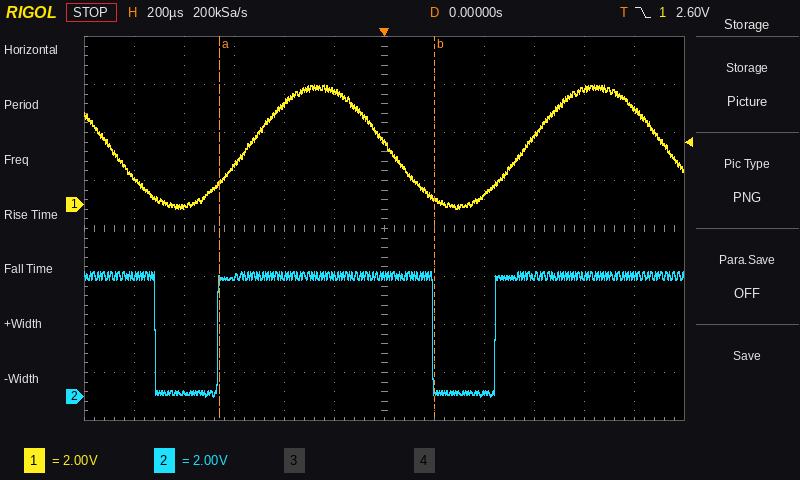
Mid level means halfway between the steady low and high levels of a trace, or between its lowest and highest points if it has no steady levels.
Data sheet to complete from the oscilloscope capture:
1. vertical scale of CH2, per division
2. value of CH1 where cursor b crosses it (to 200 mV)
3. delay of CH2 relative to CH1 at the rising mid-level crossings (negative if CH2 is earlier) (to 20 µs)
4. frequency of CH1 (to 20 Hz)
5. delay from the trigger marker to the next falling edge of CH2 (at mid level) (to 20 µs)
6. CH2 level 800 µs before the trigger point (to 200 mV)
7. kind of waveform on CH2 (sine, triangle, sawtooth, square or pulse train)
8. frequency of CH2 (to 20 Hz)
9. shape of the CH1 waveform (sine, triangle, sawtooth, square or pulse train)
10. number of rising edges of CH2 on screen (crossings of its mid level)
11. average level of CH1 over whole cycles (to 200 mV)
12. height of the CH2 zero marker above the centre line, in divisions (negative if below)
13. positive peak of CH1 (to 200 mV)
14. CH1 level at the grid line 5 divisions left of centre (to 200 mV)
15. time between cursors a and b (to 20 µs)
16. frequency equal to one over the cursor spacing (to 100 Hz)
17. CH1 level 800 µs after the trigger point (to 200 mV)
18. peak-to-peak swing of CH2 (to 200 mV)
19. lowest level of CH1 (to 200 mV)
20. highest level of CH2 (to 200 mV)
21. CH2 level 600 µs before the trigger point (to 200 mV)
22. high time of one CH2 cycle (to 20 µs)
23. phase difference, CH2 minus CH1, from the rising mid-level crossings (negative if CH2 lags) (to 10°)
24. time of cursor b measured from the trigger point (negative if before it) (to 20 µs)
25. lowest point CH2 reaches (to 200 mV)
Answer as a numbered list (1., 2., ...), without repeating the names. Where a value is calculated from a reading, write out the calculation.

1. 2 V
2. 200 mV
3. -120 µs
4. 900 Hz
5. 200 µs
6. 200 mV
7. pulse train
8. 900 Hz
9. sine
10. 2
11. (5.0 V + (-200 mV)) / 2 ≈ 2.4 V
12. -3.5 div
13. 5.0 V
14. 1.2 V
15. 860 µs
16. 1 / 860 µs ≈ 1.2 kHz
17. 4.8 V
18. 5.2 V − (0.0 V) = 5.2 V
19. -200 mV
20. 5.2 V
21. 5.0 V
22. 860 µs
23. +40°
24. +200 µs
25. 0.0 V
